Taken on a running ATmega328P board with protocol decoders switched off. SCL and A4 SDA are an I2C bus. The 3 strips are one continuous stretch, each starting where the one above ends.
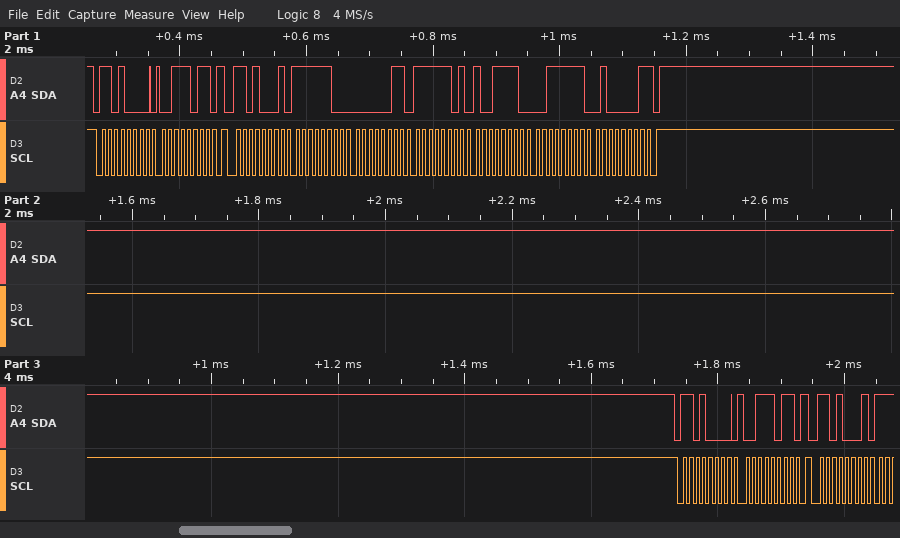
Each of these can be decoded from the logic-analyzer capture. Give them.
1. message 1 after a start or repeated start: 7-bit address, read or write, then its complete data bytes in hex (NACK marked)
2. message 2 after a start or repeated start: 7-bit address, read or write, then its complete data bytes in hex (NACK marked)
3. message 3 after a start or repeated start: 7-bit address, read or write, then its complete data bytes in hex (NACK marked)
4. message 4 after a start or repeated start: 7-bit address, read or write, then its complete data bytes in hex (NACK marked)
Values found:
0x68 write: 3B
0x68 read: FC 03 FD 9E 3F 41 NACK
0x68 write: 3B
0x68 read
